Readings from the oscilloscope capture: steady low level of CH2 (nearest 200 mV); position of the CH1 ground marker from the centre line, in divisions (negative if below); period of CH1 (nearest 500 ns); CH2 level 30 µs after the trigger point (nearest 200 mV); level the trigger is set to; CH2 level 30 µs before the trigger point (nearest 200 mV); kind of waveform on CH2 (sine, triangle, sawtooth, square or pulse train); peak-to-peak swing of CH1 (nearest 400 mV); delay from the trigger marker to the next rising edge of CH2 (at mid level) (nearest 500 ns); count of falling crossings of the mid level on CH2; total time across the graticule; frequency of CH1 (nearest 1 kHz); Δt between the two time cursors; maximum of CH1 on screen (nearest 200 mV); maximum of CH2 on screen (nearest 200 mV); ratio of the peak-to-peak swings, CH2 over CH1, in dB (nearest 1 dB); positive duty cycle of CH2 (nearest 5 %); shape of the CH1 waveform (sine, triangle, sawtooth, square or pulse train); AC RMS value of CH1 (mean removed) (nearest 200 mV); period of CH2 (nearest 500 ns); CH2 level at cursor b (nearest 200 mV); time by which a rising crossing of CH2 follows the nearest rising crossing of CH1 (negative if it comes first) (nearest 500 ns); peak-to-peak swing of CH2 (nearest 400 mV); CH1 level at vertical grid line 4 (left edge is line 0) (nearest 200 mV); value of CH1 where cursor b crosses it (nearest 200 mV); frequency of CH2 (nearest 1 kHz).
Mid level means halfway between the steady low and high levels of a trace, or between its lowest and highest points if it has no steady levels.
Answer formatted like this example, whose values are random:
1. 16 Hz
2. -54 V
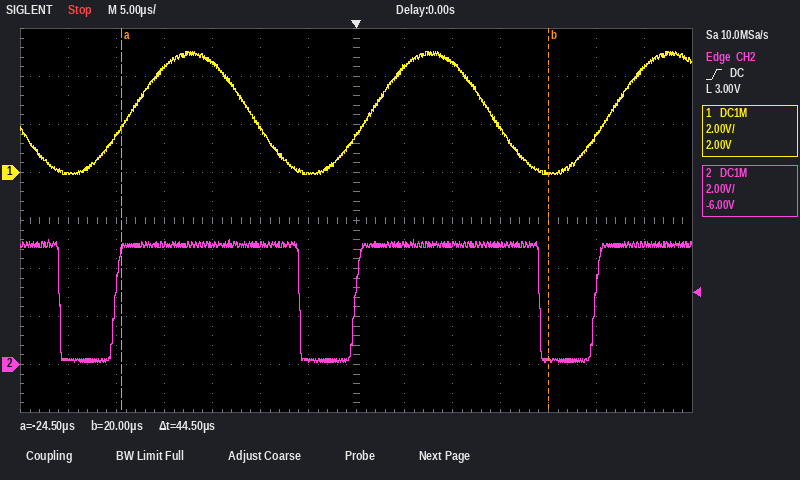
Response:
1. 200 mV
2. +1.0 div
3. 25.0 µs
4. 5.0 V
5. 3.00 V
6. 200 mV
7. pulse train
8. 5.2 V
9. 25.0 µs
10. 3
11. 70 µs
12. 40 kHz
13. 44.5 µs
14. 5.0 V
15. 5.2 V
16. 0 dB
17. 75 %
18. sine
19. 1.8 V
20. 25.0 µs
21. 200 mV
22. -1.5 µs
23. 5.2 V
24. 4.6 V
25. 0.0 V
26. 40 kHz
